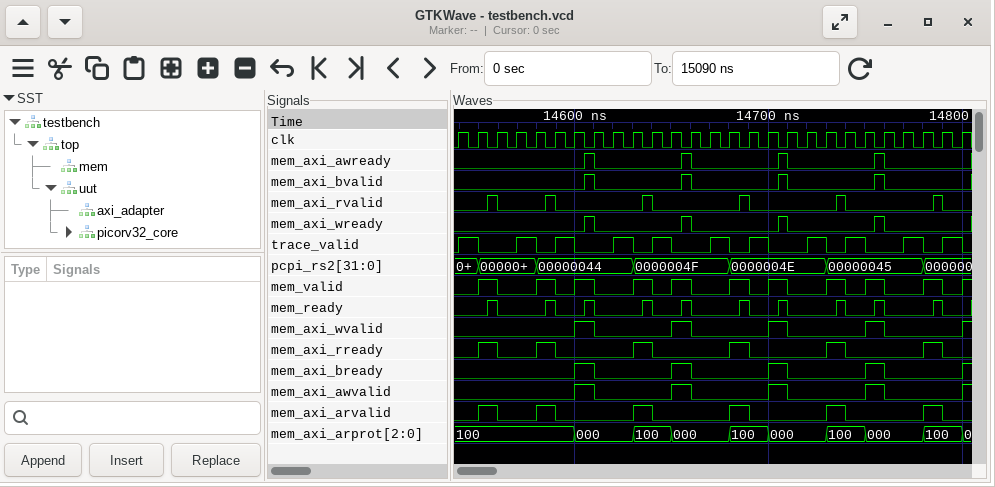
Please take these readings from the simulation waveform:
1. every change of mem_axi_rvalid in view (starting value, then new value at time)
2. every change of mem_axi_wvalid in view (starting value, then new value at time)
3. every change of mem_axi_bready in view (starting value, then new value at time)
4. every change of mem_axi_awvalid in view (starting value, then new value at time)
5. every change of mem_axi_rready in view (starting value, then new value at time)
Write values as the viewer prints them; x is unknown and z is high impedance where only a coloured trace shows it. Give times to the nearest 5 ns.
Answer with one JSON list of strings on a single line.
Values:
["0, 1 at 14555 ns, 0 at 14560 ns, 1 at 14585 ns, 0 at 14590 ns, 1 at 14635 ns, 0 at 14640 ns, 1 at 14685 ns, 0 at 14690 ns, 1 at 14735 ns, 0 at 14740 ns, 1 at 14785 ns, 0 at 14790 ns", "0, 1 at 14600 ns, 0 at 14610 ns, 1 at 14650 ns, 0 at 14660 ns, 1 at 14700 ns, 0 at 14710 ns, 1 at 14750 ns, 0 at 14760 ns, 1 at 14800 ns", "0, 1 at 14600 ns, 0 at 14610 ns, 1 at 14650 ns, 0 at 14660 ns, 1 at 14700 ns, 0 at 14710 ns, 1 at 14750 ns, 0 at 14760 ns, 1 at 14800 ns", "0, 1 at 14600 ns, 0 at 14610 ns, 1 at 14650 ns, 0 at 14660 ns, 1 at 14700 ns, 0 at 14710 ns, 1 at 14750 ns, 0 at 14760 ns, 1 at 14800 ns", "0, 1 at 14550 ns, 0 at 14560 ns, 1 at 14580 ns, 0 at 14590 ns, 1 at 14630 ns, 0 at 14640 ns, 1 at 14680 ns, 0 at 14690 ns, 1 at 14730 ns, 0 at 14740 ns, 1 at 14780 ns, 0 at 14790 ns"]
